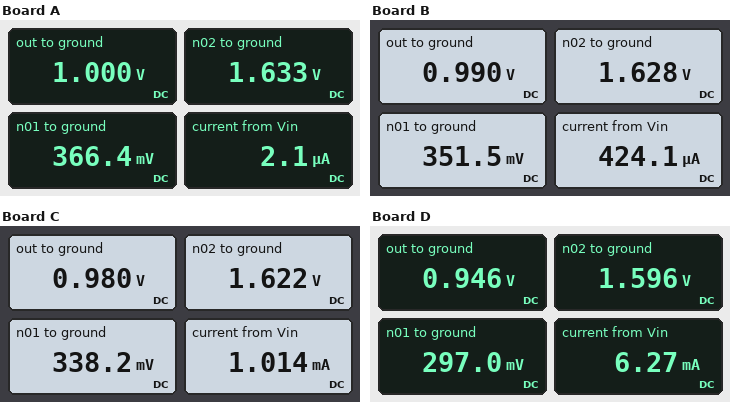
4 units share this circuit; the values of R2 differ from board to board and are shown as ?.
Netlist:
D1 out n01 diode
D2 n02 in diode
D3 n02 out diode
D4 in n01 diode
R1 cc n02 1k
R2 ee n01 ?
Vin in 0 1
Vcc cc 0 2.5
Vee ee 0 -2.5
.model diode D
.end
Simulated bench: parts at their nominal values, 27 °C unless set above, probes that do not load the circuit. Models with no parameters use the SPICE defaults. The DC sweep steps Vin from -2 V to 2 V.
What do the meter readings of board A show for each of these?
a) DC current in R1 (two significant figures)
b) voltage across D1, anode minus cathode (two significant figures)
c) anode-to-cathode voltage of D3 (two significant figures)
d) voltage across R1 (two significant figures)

870 µA
630 mV
630 mV
870 mV
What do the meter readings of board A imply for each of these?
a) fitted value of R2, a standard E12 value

3.3 kΩ
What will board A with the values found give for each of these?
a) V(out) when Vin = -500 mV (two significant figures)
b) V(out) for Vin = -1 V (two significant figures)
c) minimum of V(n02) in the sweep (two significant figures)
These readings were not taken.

-460 mV
-940 mV
-1.3 V
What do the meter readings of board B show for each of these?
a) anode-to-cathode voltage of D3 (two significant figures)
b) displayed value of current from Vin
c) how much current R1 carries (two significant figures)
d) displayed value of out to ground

640 mV
424.1 µA
870 µA
0.990 V
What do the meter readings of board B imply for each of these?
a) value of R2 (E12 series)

2.2 kΩ
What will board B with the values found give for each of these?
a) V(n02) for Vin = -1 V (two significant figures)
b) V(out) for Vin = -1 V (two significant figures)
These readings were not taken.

-320 mV
-950 mV
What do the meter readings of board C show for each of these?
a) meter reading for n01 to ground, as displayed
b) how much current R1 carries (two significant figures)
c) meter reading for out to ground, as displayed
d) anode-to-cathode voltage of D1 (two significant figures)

338.2 mV
880 µA
0.980 V
640 mV
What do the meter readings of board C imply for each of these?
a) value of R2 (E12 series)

1.5 kΩ
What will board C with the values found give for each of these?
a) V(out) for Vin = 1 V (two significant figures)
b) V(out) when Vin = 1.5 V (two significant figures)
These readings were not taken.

980 mV
1.5 V
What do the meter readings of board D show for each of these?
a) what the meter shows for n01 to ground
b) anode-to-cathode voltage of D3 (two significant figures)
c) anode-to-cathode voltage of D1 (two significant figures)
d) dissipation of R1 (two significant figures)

297.0 mV
650 mV
650 mV
820 µW
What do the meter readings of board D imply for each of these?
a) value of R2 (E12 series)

390 Ω
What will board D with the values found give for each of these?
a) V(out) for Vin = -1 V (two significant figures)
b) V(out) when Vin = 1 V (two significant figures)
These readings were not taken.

-990 mV
950 mV
